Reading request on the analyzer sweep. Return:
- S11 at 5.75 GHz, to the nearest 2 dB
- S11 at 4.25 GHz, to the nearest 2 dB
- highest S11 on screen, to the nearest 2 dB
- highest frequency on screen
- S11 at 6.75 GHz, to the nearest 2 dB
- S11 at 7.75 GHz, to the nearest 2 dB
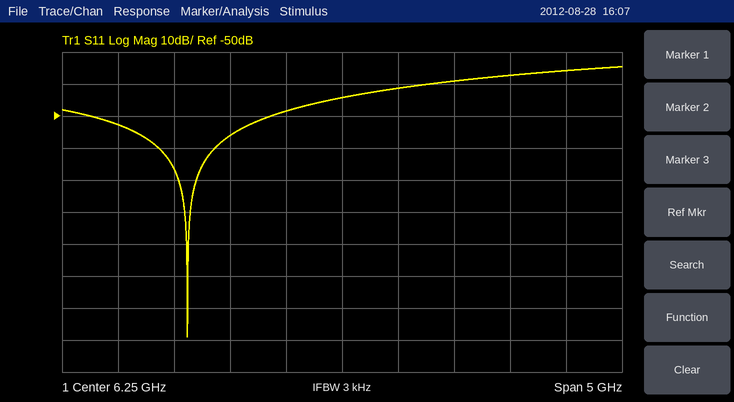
-48 dB
-52 dB
-34 dB
8.75 GHz
-42 dB
-38 dB
